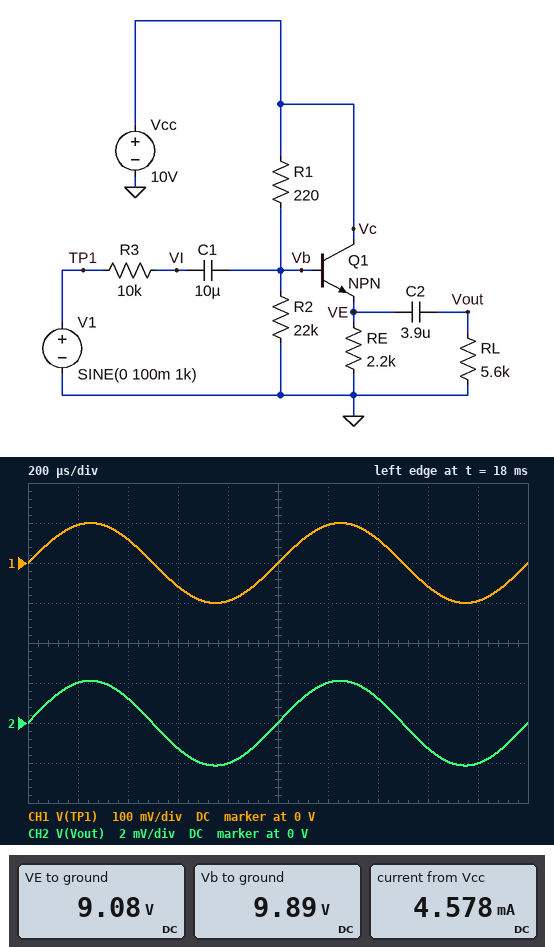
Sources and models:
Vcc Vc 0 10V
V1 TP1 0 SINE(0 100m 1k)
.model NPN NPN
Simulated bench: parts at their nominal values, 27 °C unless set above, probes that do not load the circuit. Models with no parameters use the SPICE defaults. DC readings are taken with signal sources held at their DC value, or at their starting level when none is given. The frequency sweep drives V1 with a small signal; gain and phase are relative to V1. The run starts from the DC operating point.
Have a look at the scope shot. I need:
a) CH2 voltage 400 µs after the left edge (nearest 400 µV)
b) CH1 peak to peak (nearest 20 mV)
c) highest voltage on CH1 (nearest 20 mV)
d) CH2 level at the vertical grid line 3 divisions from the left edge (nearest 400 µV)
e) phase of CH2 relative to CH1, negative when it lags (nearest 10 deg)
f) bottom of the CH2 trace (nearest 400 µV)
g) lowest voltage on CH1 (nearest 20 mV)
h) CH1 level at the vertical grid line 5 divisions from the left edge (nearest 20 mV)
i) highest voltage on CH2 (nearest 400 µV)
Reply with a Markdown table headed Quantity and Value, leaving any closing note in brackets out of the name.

| Quantity | Value |
|---|---|
| CH2 voltage 400 µs after the left edge | 1.2 mV |
| CH1 peak to peak | 200 mV |
| highest voltage on CH1 | 100 mV |
| CH2 level at the vertical grid line 3 divisions from the left edge | -1.2 mV |
| phase of CH2 relative to CH1, negative when it lags | 0 deg |
| bottom of the CH2 trace | -2.0 mV |
| lowest voltage on CH1 | -100 mV |
| CH1 level at the vertical grid line 5 divisions from the left edge | 0 V |
| highest voltage on CH2 | 2.0 mV |
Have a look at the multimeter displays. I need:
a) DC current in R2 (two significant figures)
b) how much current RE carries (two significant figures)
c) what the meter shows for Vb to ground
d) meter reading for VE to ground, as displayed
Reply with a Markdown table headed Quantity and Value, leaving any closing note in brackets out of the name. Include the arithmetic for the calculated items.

| Quantity | Value |
|---|---|
| DC current in R2 | (9.89 V) / 22 kΩ = 450 µA |
| how much current RE carries | (9.08 V) / 2.2 kΩ = 4.1 mA |
| what the meter shows for Vb to ground | 9.89 V |
| meter reading for VE to ground, as displayed | 9.08 V |
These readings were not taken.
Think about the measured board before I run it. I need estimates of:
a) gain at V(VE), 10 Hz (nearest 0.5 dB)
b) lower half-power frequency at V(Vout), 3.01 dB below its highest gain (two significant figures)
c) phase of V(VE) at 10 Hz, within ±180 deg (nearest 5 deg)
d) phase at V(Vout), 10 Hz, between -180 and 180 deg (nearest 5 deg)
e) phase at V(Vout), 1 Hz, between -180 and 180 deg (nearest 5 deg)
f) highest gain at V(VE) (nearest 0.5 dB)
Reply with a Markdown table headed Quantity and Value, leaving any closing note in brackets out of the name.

| Quantity | Value |
|---|---|
| gain at V(VE), 10 Hz | -33.5 dB |
| lower half-power frequency at V(Vout), 3.01 dB below its highest gain | 7.6 Hz |
| phase of V(VE) at 10 Hz, within ±180 deg | 10 deg |
| phase at V(Vout), 10 Hz, between -180 and 180 deg | 45 deg |
| phase at V(Vout), 1 Hz, between -180 and 180 deg | 140 deg |
| highest gain at V(VE) | -33.5 dB |
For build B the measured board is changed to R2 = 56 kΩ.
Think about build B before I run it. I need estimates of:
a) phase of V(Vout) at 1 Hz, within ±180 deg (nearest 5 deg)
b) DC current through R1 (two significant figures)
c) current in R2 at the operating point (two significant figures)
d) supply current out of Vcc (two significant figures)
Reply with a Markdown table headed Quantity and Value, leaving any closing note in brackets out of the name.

| Quantity | Value |
|---|---|
| phase of V(Vout) at 1 Hz, within ±180 deg | 140 deg |
| DC current through R1 | 220 µA |
| current in R2 at the operating point | 180 µA |
| supply current out of Vcc | 4.3 mA |
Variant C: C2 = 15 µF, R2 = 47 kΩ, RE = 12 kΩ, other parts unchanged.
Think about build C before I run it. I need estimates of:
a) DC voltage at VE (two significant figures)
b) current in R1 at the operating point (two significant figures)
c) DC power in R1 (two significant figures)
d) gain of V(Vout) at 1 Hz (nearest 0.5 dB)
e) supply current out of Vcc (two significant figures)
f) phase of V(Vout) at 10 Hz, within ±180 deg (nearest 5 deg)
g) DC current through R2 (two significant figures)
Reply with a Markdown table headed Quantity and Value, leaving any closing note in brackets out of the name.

| Quantity | Value |
|---|---|
| DC voltage at VE | 9.2 V |
| current in R1 at the operating point | 220 µA |
| DC power in R1 | 11 µW |
| gain of V(Vout) at 1 Hz | -45.5 dB |
| supply current out of Vcc | 980 µA |
| phase of V(Vout) at 10 Hz, within ±180 deg | 20 deg |
| DC current through R2 | 210 µA |
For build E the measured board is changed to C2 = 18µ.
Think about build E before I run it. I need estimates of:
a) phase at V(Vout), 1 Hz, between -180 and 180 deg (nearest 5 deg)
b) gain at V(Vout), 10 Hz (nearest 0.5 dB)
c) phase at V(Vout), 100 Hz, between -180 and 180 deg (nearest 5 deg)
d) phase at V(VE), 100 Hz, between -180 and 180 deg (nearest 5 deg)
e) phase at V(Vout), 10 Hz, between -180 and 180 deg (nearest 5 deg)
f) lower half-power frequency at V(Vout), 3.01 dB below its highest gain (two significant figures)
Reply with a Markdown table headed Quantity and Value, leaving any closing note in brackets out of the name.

| Quantity | Value |
|---|---|
| phase at V(Vout), 1 Hz, between -180 and 180 deg | 115 deg |
| gain at V(Vout), 10 Hz | -33.5 dB |
| phase at V(Vout), 100 Hz, between -180 and 180 deg | 0 deg |
| phase at V(VE), 100 Hz, between -180 and 180 deg | 0 deg |
| phase at V(Vout), 10 Hz, between -180 and 180 deg | 20 deg |
| lower half-power frequency at V(Vout), 3.01 dB below its highest gain | 2.4 Hz |
